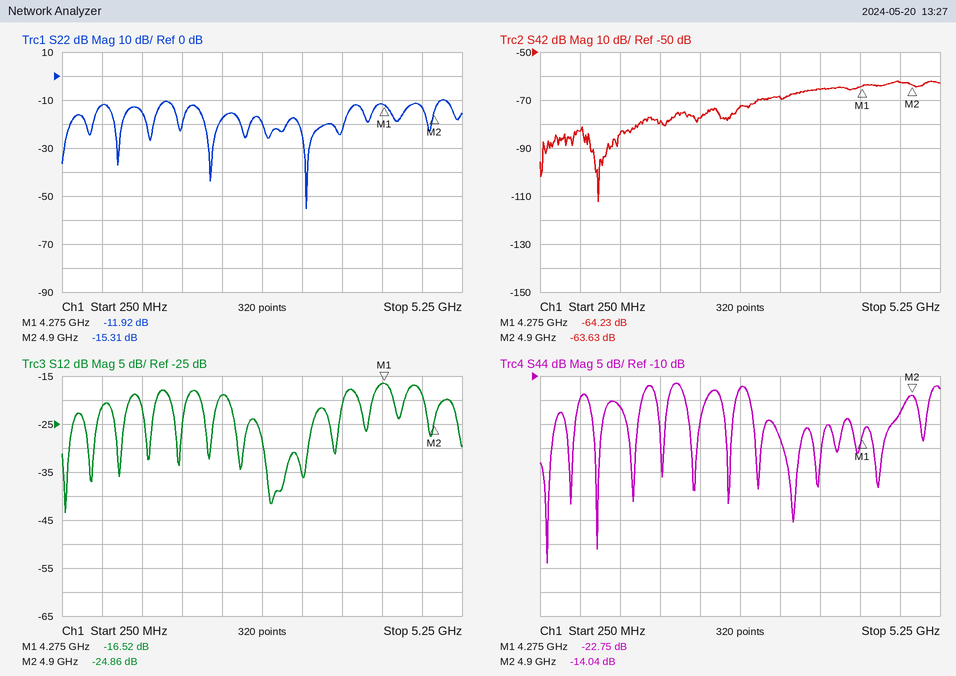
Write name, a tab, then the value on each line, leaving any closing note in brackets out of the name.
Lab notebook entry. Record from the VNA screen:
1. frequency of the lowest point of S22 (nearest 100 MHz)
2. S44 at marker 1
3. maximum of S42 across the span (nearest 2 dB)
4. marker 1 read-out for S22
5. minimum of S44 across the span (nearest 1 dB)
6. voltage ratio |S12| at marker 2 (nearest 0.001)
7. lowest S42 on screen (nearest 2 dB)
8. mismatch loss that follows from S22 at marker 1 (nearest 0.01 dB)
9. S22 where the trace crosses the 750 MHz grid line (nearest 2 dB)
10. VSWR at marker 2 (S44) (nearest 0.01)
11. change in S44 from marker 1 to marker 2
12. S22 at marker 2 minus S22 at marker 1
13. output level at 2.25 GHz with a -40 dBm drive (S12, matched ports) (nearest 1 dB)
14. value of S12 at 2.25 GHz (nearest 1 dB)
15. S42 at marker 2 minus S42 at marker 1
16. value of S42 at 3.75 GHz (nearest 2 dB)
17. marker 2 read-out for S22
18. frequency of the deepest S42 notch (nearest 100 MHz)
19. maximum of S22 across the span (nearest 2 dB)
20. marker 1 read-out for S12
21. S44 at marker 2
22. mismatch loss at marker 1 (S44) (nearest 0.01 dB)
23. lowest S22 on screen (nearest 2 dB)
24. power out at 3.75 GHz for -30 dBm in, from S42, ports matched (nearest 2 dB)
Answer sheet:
frequency of the lowest point of S22	3.3 GHz
S44 at marker 1	-22.75 dB
maximum of S42 across the span	-62 dB
marker 1 read-out for S22	-11.92 dB
minimum of S44 across the span	-49 dB
voltage ratio |S12| at marker 2	0.057
lowest S42 on screen	-112 dB
mismatch loss that follows from S22 at marker 1	0.29 dB
S22 where the trace crosses the 750 MHz grid line	-12 dB
VSWR at marker 2 (S44)	1.50
change in S44 from marker 1 to marker 2	8.71 dB
S22 at marker 2 minus S22 at marker 1	-3.39 dB
output level at 2.25 GHz with a -40 dBm drive (S12, matched ports)	-59 dBm
value of S12 at 2.25 GHz	-19 dB
S42 at marker 2 minus S42 at marker 1	0.60 dB
value of S42 at 3.75 GHz	-66 dB
marker 2 read-out for S22	-15.31 dB
frequency of the deepest S42 notch	1.0 GHz
maximum of S22 across the span	-10 dB
marker 1 read-out for S12	-16.52 dB
S44 at marker 2	-14.04 dB
mismatch loss at marker 1 (S44)	0.02 dB
lowest S22 on screen	-56 dB
power out at 3.75 GHz for -30 dBm in, from S42, ports matched	-96 dBm
